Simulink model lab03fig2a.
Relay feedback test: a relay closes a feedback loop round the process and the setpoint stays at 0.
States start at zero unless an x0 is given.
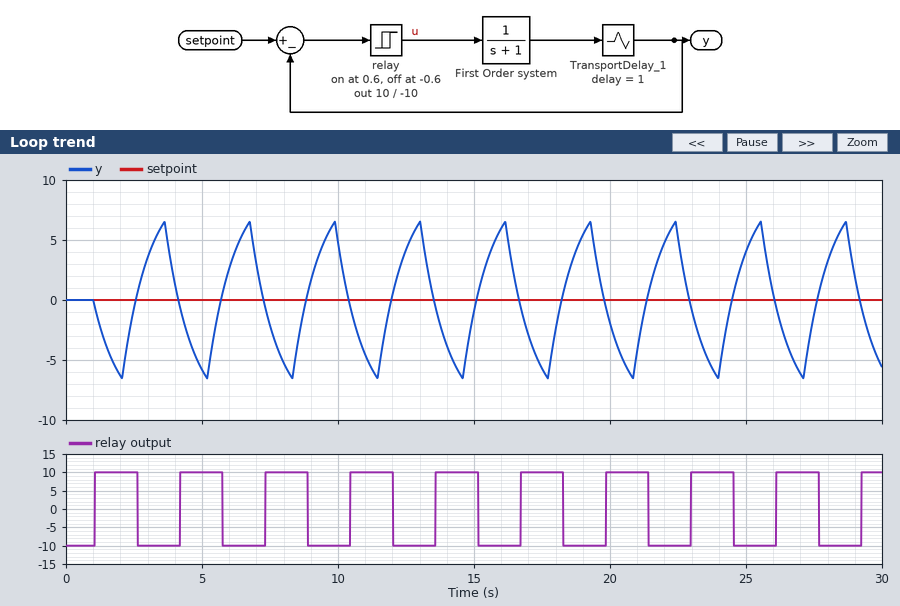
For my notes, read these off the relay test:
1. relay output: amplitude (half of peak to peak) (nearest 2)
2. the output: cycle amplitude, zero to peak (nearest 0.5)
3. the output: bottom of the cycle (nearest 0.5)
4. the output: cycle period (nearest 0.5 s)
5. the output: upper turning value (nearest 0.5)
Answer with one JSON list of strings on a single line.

["10", "6.5", "-6.5", "3.0 s", "6.5"]
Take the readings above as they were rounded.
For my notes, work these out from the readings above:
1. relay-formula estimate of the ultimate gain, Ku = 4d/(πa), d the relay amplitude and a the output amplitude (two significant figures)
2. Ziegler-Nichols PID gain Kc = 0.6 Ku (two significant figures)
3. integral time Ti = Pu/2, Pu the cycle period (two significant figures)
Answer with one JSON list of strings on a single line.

["2.0", "1.2", "1.5 s"]
